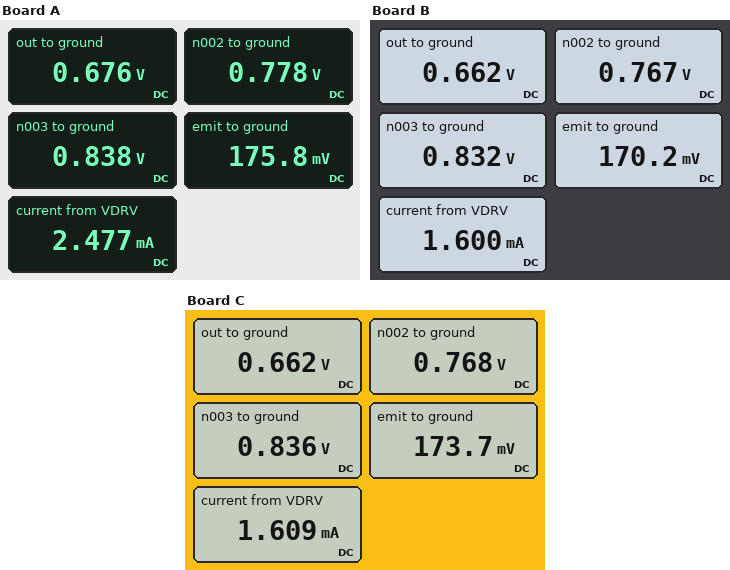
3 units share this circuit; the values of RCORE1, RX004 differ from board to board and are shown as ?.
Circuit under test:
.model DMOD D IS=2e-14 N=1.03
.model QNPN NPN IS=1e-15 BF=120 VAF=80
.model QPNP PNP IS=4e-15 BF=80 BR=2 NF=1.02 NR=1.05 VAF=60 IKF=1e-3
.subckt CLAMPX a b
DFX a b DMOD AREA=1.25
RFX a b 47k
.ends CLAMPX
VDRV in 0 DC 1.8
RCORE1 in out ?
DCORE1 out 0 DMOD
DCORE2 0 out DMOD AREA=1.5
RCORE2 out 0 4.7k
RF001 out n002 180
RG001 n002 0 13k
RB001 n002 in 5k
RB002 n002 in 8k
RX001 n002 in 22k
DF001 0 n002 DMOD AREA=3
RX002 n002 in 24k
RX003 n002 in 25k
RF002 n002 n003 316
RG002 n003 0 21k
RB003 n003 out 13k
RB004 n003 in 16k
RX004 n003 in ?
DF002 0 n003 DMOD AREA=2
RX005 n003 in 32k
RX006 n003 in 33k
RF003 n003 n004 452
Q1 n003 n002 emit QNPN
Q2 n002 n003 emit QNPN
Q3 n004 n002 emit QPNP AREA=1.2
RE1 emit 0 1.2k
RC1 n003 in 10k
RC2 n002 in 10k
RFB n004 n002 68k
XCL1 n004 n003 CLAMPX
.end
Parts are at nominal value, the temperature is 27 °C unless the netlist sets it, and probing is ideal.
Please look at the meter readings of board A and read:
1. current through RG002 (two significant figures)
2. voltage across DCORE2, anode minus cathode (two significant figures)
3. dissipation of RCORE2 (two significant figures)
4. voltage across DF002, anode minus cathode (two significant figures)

40 µA
-680 mV
97 µW
-840 mV
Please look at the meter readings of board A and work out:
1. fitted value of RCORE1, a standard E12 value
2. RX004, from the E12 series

680 Ω
22 kΩ
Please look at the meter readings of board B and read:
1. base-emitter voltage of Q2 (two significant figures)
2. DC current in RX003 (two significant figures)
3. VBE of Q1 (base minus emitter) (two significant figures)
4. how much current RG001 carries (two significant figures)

660 mV
41 µA
600 mV
59 µA
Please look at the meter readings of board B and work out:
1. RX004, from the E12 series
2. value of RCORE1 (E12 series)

18 kΩ
1.5 kΩ
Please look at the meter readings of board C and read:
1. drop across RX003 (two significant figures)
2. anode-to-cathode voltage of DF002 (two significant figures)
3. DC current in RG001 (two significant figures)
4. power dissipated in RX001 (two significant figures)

1.0 V
-840 mV
59 µA
48 µW
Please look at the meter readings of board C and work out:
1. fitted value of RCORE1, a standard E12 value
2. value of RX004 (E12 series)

1.5 kΩ
15 kΩ
